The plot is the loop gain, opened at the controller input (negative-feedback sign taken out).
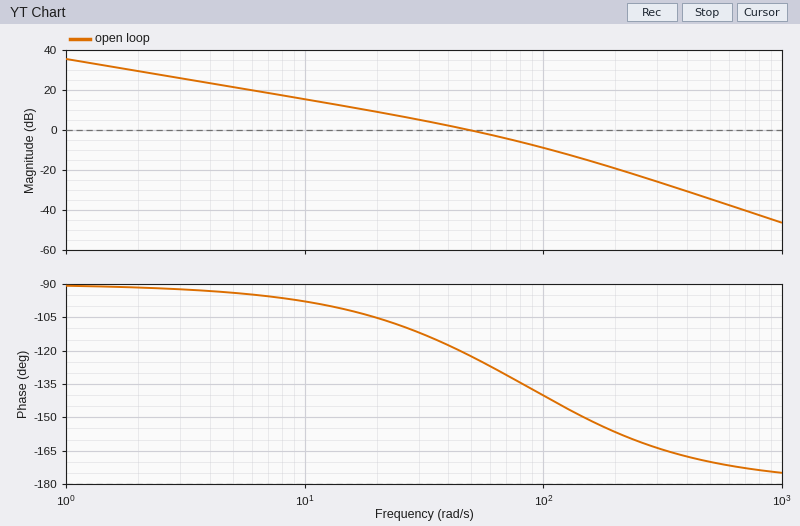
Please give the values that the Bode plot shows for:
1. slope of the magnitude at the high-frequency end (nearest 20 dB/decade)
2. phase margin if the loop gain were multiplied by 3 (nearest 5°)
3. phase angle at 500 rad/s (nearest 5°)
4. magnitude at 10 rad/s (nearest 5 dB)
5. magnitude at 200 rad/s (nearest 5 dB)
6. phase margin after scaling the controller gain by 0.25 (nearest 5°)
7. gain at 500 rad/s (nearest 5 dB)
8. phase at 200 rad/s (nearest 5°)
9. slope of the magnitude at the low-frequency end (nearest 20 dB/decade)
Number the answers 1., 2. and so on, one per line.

1. -40 dB/decade
2. 40°
3. -170°
4. 15 dB
5. -20 dB
6. 80°
7. -35 dB
8. -155°
9. -20 dB/decade
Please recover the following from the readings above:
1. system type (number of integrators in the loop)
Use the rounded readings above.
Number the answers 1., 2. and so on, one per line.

1. 1
